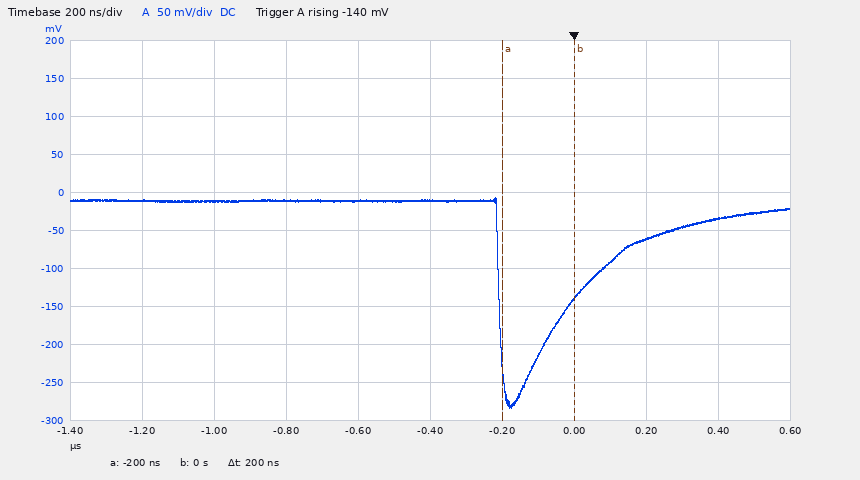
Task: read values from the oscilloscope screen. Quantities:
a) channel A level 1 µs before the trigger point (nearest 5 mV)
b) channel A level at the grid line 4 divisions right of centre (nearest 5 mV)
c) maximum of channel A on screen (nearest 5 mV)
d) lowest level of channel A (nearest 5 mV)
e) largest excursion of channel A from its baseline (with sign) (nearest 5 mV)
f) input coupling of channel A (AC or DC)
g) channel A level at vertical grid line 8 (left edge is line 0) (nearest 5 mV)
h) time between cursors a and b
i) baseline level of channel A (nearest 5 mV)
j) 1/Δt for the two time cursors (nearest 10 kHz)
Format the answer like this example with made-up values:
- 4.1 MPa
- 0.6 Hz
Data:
- -10 mV
- -35 mV
- -5 mV
- -285 mV
- -275 mV
- DC
- -60 mV
- 200 ns
- -10 mV
- 5.00 MHz
